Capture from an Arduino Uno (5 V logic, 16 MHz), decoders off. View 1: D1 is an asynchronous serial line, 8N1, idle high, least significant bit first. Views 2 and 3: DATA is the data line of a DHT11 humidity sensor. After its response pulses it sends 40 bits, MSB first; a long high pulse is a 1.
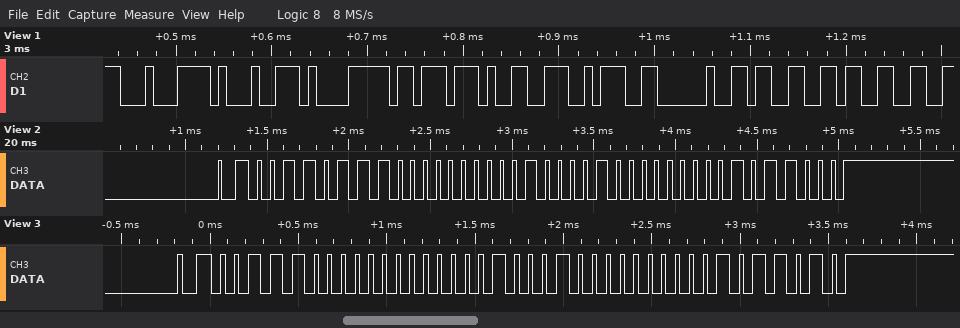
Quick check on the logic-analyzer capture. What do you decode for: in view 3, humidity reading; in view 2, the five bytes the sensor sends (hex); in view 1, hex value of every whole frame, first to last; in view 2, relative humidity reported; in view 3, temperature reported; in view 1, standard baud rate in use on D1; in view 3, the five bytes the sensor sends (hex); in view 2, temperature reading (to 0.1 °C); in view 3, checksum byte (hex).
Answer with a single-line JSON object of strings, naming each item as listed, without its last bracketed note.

{"in view 3, humidity reading": "56 %", "in view 2, the five bytes the sensor sends": "37 00 21 00 58", "in view 1, hex value of every whole frame, first to last": "0xC4 0x91 0xE1 0xBB 0x99 0x3A 0x20 0x33 0x33", "in view 2, relative humidity reported": "55 %", "in view 3, temperature reported": "34.0 °C", "in view 1, standard baud rate in use on D1": "115200 baud", "in view 3, the five bytes the sensor sends": "38 00 22 00 5A", "in view 2, temperature reading": "33.0 °C", "in view 3, checksum byte": "0x5A"}
